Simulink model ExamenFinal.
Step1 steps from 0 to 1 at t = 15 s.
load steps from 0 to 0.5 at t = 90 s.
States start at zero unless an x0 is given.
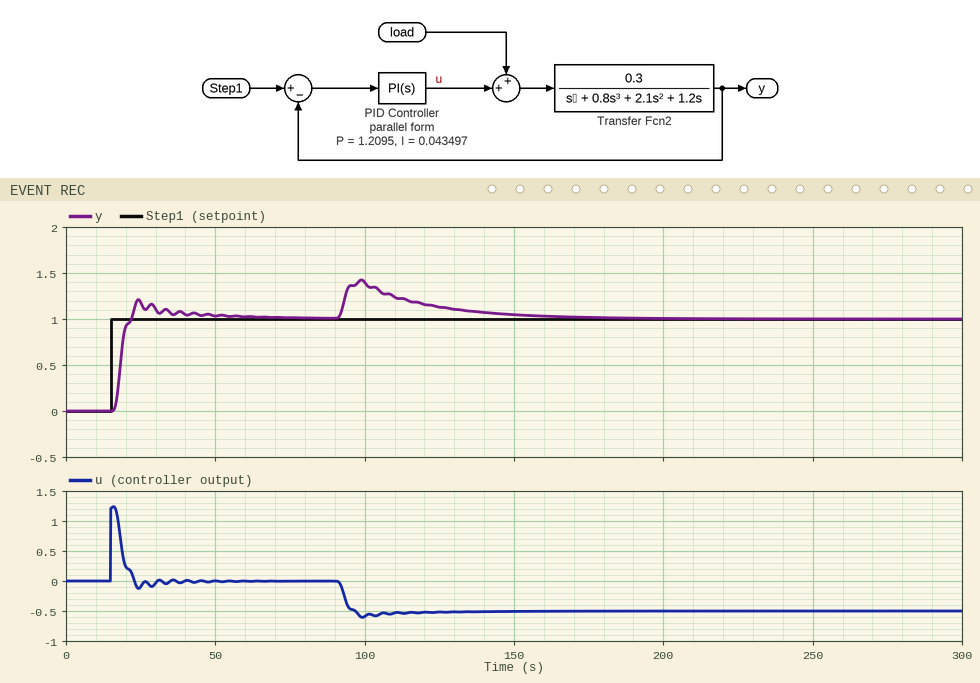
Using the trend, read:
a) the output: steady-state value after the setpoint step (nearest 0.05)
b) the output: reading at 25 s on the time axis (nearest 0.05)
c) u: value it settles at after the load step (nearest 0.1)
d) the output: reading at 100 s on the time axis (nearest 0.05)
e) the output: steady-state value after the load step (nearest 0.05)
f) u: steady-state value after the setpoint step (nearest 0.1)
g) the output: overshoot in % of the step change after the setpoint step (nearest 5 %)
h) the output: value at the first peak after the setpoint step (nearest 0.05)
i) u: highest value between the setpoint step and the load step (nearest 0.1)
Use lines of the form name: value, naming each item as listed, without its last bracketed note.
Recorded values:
the output: steady-state value after the setpoint step: 1.00
the output: reading at 25 s on the time axis: 1.20
u: value it settles at after the load step: -0.5
the output: reading at 100 s on the time axis: 1.40
the output: steady-state value after the load step: 1.00
u: steady-state value after the setpoint step: 0.0
the output: overshoot in % of the step change after the setpoint step: 20 %
the output: value at the first peak after the setpoint step: 1.20
u: highest value between the setpoint step and the load step: 1.2
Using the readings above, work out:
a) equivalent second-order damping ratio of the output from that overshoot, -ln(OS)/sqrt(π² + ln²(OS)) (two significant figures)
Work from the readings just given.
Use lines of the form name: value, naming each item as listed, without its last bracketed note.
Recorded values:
equivalent second-order damping ratio of the output from that overshoot, -ln(OS)/sqrt(π² + ln²(OS)): 0.46
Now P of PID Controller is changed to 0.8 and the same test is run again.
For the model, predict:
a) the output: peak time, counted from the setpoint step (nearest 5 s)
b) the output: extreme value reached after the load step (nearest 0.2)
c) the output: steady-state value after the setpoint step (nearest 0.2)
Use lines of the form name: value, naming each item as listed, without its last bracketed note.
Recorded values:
the output: peak time, counted from the setpoint step: 15 s
the output: extreme value reached after the load step: 1.6
the output: steady-state value after the setpoint step: 1.0
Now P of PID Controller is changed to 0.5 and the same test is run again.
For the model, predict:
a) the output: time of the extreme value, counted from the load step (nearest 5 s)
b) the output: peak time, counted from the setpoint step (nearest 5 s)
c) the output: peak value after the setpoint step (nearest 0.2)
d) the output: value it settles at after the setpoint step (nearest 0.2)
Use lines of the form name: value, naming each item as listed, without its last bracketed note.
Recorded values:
the output: time of the extreme value, counted from the load step: 15 s
the output: peak time, counted from the setpoint step: 20 s
the output: peak value after the setpoint step: 1.4
the output: value it settles at after the setpoint step: 1.0
